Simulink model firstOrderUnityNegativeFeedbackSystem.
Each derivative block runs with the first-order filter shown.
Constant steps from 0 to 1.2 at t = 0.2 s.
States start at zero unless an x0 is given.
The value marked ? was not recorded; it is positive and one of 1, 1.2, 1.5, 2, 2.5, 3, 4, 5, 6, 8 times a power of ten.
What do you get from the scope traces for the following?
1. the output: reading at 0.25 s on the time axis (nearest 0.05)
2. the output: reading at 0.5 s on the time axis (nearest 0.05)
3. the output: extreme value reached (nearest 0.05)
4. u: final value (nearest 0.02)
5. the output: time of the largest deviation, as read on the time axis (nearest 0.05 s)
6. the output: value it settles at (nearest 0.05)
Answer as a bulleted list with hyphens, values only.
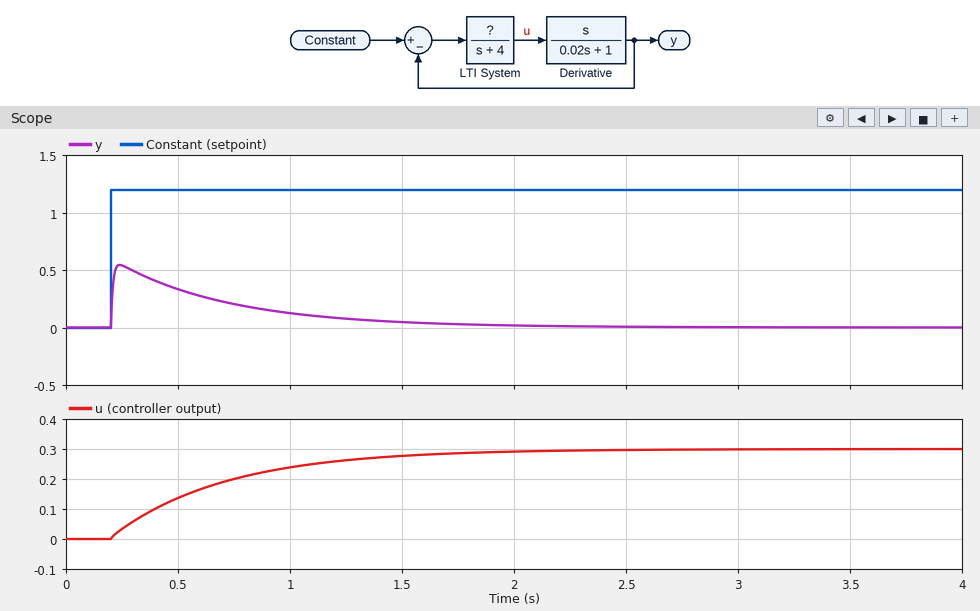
- 0.55
- 0.35
- 0.55
- 0.30
- 0.25 s
- 0.00
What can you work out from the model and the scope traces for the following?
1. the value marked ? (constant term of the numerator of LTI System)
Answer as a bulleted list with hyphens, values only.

- 1
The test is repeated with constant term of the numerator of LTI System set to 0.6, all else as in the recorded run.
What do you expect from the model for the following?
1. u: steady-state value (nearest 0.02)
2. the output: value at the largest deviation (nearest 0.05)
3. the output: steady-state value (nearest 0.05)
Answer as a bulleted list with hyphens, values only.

- 0.18
- 0.40
- 0.00
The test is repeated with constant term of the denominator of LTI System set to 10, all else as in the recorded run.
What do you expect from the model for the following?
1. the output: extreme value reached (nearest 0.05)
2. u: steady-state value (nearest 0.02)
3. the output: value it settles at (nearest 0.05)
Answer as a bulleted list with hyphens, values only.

- 0.50
- 0.12
- 0.00
